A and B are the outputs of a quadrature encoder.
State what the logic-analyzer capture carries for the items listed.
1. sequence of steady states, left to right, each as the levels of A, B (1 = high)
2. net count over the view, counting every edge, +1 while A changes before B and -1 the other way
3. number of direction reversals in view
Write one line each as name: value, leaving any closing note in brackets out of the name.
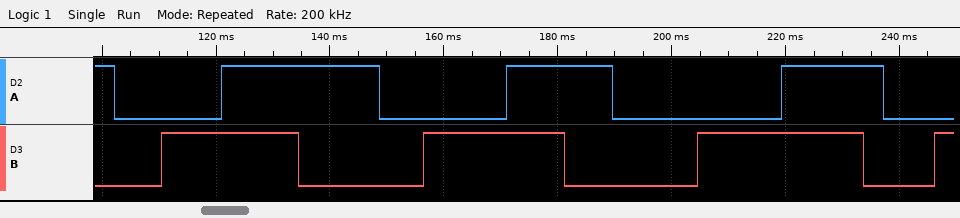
sequence of steady states, left to right, each as the levels of A, B: 10 00 01 11 10 00 01 11 10 00 01 11 10 00 01
net count over the view, counting every edge, +1 while A changes before B and -1 the other way: -14
number of direction reversals in view: 0
